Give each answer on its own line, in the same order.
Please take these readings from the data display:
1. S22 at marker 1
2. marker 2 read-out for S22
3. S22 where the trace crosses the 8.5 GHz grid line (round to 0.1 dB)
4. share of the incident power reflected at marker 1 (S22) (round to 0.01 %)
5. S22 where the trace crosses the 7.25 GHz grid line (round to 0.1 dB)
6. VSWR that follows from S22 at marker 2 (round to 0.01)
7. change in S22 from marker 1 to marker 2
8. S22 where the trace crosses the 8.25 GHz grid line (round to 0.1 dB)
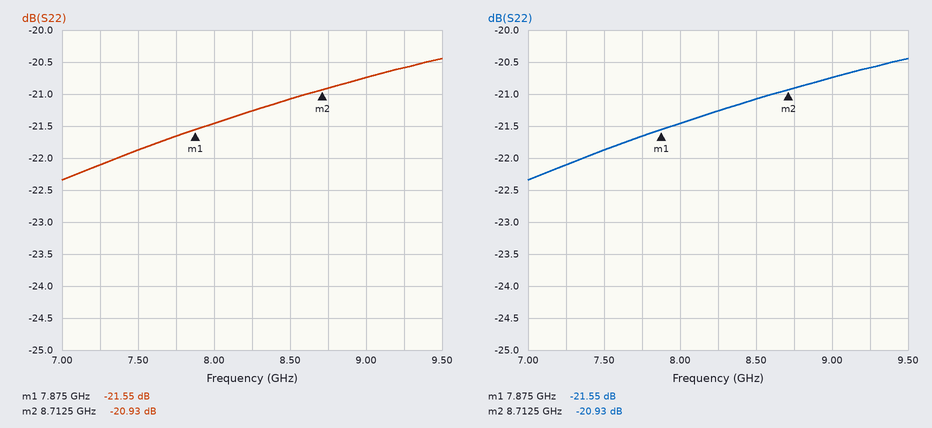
-21.55 dB
-20.93 dB
-21.1 dB
0.70 %
-22.1 dB
1.20
0.62 dB
-21.3 dB
